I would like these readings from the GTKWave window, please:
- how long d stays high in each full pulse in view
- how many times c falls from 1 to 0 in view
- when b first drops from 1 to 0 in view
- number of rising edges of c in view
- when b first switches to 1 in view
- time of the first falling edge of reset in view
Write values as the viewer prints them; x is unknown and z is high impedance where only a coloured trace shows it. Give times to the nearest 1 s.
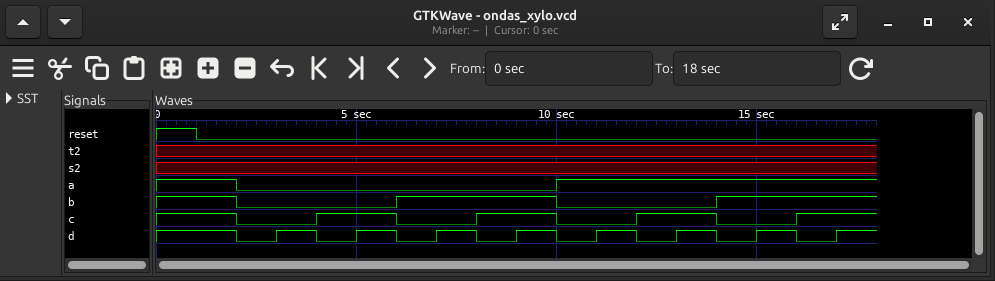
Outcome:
1 s, 1 s, 1 s, 1 s, 1 s, 1 s, 1 s
4
2 s
4
6 s
1 s
